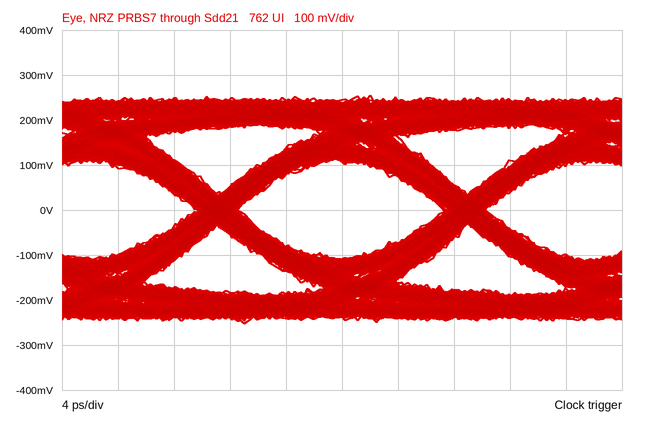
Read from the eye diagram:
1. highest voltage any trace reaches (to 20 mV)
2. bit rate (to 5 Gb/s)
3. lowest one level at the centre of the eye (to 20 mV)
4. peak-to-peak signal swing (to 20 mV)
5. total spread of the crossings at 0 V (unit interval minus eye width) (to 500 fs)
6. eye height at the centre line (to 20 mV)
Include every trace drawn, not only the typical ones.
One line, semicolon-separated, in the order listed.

260 mV; 55 Gb/s; 100 mV; 500 mV; 3.0 ps; 220 mV
